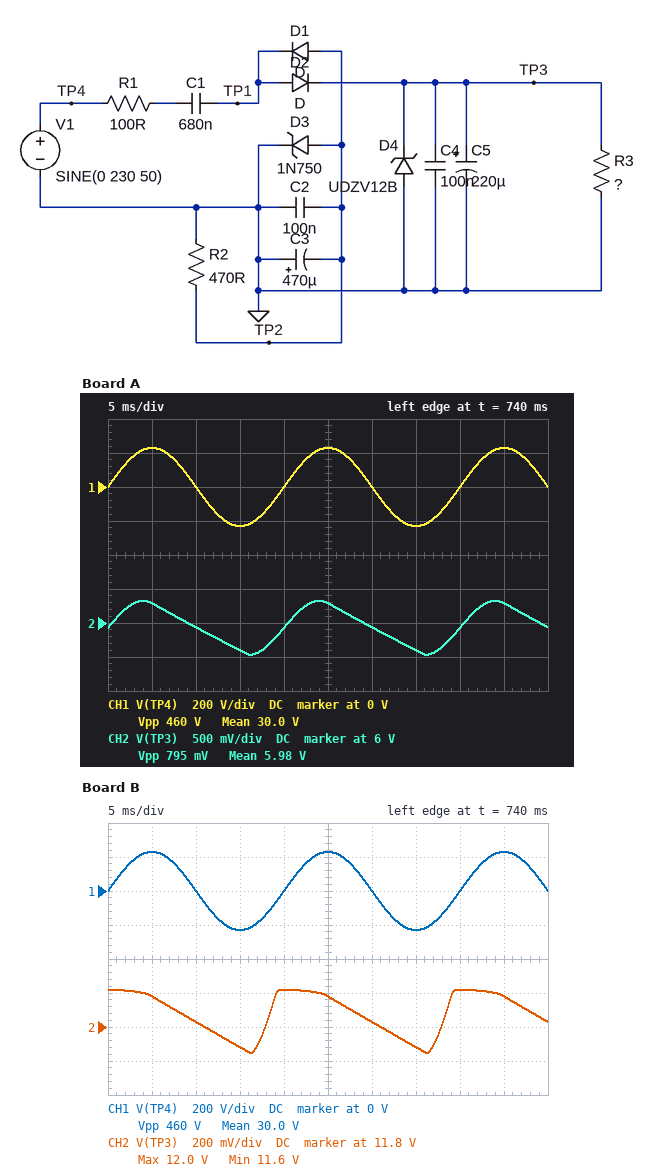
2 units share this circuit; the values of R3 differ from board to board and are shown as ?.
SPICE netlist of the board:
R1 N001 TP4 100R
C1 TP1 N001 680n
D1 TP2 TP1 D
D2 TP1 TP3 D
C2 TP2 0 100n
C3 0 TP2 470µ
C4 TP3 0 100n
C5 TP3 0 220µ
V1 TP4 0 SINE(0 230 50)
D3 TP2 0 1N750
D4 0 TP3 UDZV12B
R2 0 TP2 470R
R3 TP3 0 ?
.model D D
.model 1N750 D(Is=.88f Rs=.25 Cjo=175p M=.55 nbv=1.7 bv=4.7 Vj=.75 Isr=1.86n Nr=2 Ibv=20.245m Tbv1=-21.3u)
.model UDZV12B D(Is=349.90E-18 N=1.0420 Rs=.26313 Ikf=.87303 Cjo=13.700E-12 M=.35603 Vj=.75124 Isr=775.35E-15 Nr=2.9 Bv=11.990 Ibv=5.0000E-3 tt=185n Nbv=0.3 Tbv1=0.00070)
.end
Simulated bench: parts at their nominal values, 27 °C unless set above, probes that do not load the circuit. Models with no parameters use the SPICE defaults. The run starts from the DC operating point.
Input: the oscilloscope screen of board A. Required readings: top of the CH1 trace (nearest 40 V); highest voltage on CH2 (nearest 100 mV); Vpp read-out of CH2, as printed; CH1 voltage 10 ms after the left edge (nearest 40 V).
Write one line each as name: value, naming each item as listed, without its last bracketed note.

top of the CH1 trace: 240 V
highest voltage on CH2: 6.3 V
Vpp read-out of CH2, as printed: 795 mV
CH1 voltage 10 ms after the left edge: 0 V
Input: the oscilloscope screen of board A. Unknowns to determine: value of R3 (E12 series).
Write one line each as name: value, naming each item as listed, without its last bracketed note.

value of R3: 390 Ω
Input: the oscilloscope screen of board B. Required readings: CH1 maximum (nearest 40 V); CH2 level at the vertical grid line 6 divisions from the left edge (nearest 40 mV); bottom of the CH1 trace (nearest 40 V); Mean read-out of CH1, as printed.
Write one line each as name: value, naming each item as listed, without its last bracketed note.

CH1 maximum: 240 V
CH2 level at the vertical grid line 6 divisions from the left edge: 11.84 V
bottom of the CH1 trace: -240 V
Mean read-out of CH1, as printed: 30.0 V
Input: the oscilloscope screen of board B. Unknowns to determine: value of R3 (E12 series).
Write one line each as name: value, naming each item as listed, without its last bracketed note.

value of R3: 1.8 kΩ
